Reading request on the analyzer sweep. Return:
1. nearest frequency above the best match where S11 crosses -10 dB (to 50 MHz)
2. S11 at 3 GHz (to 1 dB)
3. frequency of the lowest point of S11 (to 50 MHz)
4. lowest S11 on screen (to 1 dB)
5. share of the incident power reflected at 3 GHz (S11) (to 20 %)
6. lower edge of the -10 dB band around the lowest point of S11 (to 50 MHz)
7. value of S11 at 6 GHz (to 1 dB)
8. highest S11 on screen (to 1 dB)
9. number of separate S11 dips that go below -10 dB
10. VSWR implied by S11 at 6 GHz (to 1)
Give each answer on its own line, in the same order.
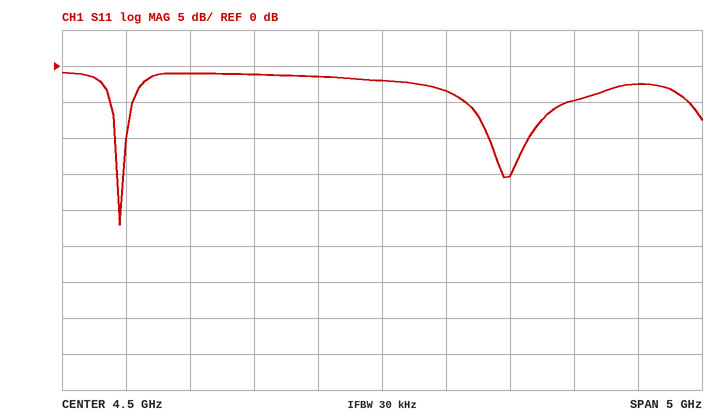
2.50 GHz
-1 dB
2.45 GHz
-22 dB
80 %
2.40 GHz
-5 dB
-1 dB
2
4
